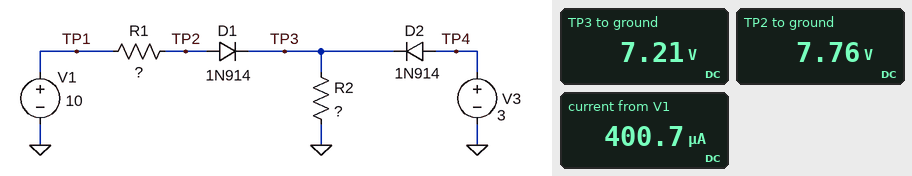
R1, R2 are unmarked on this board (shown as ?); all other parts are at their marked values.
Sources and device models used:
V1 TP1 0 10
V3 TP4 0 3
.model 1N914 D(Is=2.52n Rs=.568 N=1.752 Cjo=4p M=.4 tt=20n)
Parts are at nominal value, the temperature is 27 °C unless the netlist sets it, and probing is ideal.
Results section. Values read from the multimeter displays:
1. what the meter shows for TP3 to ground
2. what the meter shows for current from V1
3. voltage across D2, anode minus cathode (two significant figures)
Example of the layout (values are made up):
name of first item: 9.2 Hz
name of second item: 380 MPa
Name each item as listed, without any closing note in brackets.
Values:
what the meter shows for TP3 to ground: 7.21 V
what the meter shows for current from V1: 400.7 µA
voltage across D2, anode minus cathode: -4.2 V
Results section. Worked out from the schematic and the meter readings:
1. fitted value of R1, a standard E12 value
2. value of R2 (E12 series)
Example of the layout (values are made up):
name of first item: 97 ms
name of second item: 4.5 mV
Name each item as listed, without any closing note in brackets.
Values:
fitted value of R1, a standard E12 value: 5.6 kΩ
value of R2: 18 kΩ
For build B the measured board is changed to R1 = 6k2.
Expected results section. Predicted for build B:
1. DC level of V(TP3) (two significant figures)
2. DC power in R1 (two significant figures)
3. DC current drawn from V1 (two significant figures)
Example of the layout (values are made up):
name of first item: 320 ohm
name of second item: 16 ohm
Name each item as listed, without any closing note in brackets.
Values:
DC level of V(TP3): 7.0 V
DC power in R1: 950 µW
DC current drawn from V1: 390 µA
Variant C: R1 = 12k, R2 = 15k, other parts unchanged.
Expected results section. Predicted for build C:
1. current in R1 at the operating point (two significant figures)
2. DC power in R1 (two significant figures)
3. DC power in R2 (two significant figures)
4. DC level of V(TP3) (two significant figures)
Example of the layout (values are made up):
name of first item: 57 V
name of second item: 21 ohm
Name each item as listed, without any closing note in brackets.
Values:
current in R1 at the operating point: 350 µA
DC power in R1: 1.5 mW
DC power in R2: 1.8 mW
DC level of V(TP3): 5.3 V
